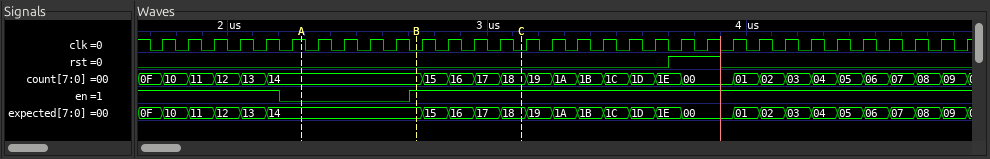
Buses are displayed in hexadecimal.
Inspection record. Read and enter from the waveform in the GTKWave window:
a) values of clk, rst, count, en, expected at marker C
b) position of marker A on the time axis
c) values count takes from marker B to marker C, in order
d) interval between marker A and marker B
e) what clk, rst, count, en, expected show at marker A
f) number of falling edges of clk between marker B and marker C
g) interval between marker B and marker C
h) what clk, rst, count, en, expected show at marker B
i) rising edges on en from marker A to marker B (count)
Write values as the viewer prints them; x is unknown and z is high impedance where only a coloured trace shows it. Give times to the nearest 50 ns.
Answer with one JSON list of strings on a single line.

["clk=0, rst=0, count=18, en=1, expected=18", "2300 ns", "14, 15, 16, 17, 18", "450 ns", "clk=1, rst=0, count=14, en=0, expected=14", "4", "400 ns", "clk=0, rst=0, count=14, en=1, expected=14", "1"]
